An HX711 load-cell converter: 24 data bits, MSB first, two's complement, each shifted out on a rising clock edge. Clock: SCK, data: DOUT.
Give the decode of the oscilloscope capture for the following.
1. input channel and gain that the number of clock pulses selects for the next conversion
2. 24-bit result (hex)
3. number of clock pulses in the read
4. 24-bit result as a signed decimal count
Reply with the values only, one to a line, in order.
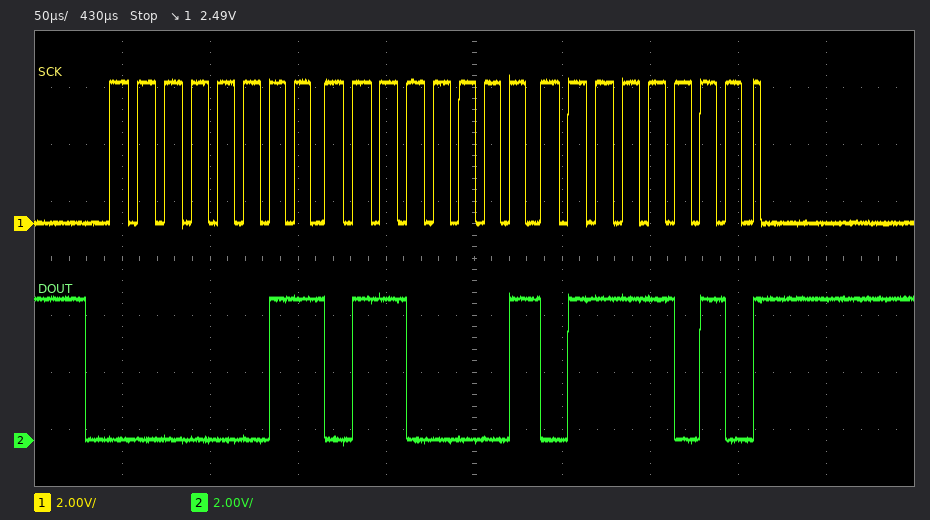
channel A, gain 128
0x03617A
25
221562
